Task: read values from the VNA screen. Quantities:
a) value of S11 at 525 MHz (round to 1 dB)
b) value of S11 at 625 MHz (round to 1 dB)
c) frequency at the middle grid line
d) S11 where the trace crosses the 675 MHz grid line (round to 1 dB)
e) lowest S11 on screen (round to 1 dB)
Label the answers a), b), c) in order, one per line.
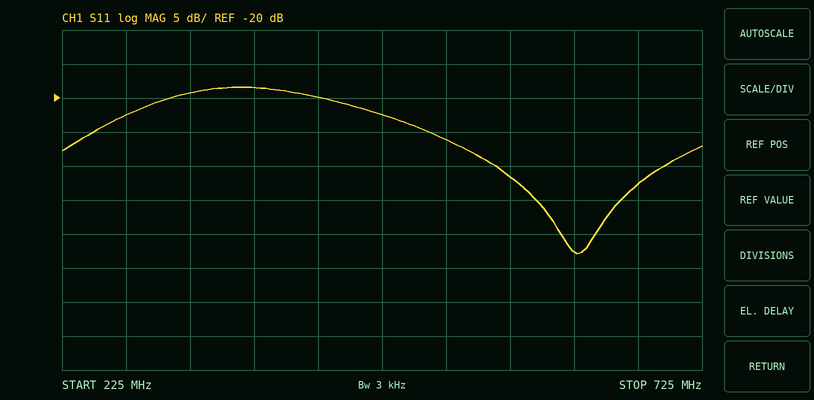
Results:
a) -26 dB
b) -43 dB
c) 475 MHz
d) -33 dB
e) -43 dB
